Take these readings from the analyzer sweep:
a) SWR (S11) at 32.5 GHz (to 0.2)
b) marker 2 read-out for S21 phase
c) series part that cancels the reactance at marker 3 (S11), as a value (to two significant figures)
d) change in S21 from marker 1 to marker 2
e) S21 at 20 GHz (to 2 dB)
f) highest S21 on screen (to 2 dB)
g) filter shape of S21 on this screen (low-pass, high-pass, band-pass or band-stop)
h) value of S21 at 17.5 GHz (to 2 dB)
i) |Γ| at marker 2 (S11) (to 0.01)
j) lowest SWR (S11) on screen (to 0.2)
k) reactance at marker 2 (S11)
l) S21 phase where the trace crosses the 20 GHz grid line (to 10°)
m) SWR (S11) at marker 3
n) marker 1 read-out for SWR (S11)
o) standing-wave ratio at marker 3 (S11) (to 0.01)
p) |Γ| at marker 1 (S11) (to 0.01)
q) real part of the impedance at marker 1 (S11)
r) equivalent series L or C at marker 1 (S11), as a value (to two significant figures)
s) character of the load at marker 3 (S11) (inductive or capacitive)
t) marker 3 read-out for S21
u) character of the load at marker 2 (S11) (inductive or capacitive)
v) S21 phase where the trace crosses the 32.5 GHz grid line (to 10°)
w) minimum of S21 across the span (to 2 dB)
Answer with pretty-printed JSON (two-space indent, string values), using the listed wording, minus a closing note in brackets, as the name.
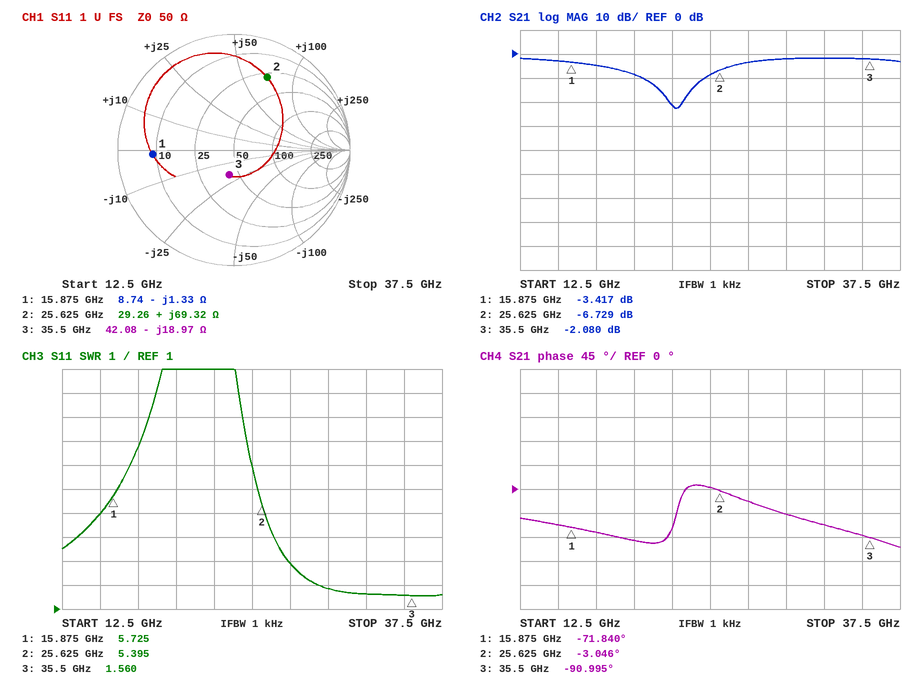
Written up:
{
  "SWR (S11) at 32.5 GHz": "1.6",
  "marker 2 read-out for S21 phase": "-3.046°",
  "series part that cancels the reactance at marker 3 (S11), as a value": "85 pH",
  "change in S21 from marker 1 to marker 2": "-3.312 dB",
  "S21 at 20 GHz": "-8 dB",
  "highest S21 on screen": "-2 dB",
  "filter shape of S21 on this screen": "band-stop",
  "value of S21 at 17.5 GHz": "-4 dB",
  "|Γ| at marker 2 (S11)": "0.69",
  "lowest SWR (S11) on screen": "1.6",
  "reactance at marker 2": "+69.32 Ω",
  "S21 phase where the trace crosses the 20 GHz grid line": "-100°",
  "SWR (S11) at marker 3": "1.560",
  "marker 1 read-out for SWR": "5.725",
  "standing-wave ratio at marker 3 (S11)": "1.56",
  "|Γ| at marker 1 (S11)": "0.70",
  "real part of the impedance at marker 1": "8.74 Ω",
  "equivalent series L or C at marker 1 (S11), as a value": "7.5 pF",
  "character of the load at marker 3 (S11)": "capacitive",
  "marker 3 read-out for S21": "-2.080 dB",
  "character of the load at marker 2 (S11)": "inductive",
  "S21 phase where the trace crosses the 32.5 GHz grid line": "-70°",
  "minimum of S21 across the span": "-22 dB"
}
